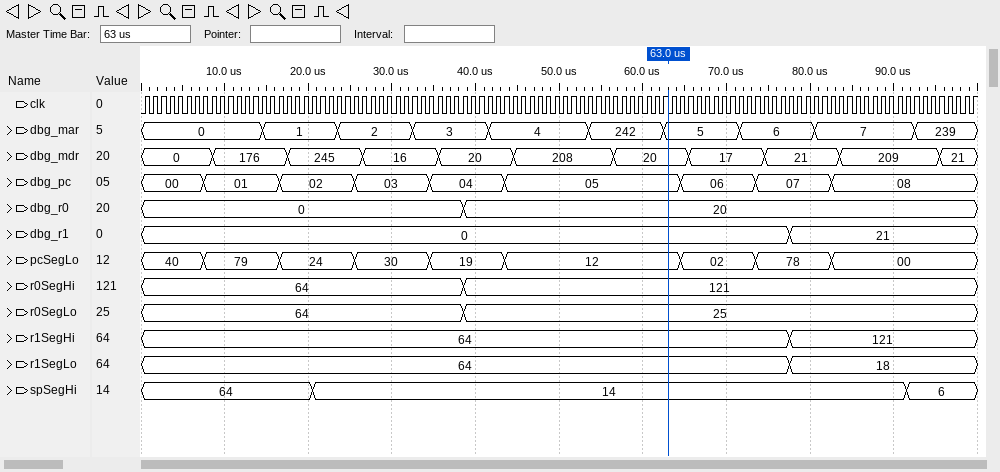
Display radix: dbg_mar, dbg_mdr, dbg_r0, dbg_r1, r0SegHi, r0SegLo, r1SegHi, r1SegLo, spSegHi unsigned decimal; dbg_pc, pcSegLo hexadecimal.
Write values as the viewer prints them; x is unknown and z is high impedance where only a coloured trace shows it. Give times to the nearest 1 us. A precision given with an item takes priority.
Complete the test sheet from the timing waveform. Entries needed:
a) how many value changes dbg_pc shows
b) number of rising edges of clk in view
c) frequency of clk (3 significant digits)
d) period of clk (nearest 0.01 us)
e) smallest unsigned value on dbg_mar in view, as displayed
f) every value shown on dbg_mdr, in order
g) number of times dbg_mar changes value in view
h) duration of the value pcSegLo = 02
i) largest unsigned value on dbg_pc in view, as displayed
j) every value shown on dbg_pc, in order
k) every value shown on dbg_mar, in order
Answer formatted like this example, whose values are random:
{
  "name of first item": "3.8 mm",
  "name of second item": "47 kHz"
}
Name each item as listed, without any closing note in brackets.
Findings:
{
  "how many value changes dbg_pc shows": "8",
  "number of rising edges of clk in view": "100",
  "frequency of clk": "1.00 MHz",
  "period of clk": "1 us",
  "smallest unsigned value on dbg_mar in view, as displayed": "0",
  "every value shown on dbg_mdr, in order": "0, 176, 245, 16, 20, 208, 20, 17, 21, 209, 21",
  "number of times dbg_mar changes value in view": "9",
  "duration of the value pcSegLo = 02": "9 us",
  "largest unsigned value on dbg_pc in view, as displayed": "08",
  "every value shown on dbg_pc, in order": "00, 01, 02, 03, 04, 05, 06, 07, 08",
  "every value shown on dbg_mar, in order": "0, 1, 2, 3, 4, 242, 5, 6, 7, 239"
}
